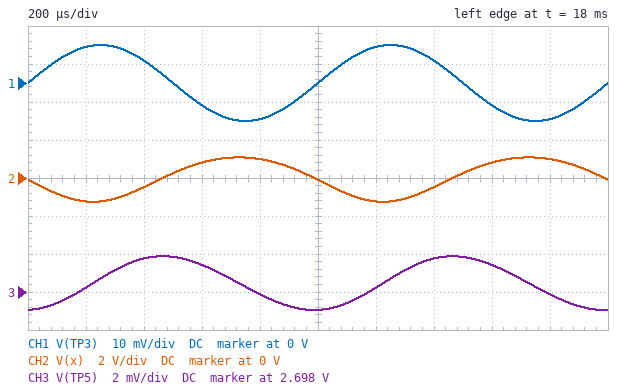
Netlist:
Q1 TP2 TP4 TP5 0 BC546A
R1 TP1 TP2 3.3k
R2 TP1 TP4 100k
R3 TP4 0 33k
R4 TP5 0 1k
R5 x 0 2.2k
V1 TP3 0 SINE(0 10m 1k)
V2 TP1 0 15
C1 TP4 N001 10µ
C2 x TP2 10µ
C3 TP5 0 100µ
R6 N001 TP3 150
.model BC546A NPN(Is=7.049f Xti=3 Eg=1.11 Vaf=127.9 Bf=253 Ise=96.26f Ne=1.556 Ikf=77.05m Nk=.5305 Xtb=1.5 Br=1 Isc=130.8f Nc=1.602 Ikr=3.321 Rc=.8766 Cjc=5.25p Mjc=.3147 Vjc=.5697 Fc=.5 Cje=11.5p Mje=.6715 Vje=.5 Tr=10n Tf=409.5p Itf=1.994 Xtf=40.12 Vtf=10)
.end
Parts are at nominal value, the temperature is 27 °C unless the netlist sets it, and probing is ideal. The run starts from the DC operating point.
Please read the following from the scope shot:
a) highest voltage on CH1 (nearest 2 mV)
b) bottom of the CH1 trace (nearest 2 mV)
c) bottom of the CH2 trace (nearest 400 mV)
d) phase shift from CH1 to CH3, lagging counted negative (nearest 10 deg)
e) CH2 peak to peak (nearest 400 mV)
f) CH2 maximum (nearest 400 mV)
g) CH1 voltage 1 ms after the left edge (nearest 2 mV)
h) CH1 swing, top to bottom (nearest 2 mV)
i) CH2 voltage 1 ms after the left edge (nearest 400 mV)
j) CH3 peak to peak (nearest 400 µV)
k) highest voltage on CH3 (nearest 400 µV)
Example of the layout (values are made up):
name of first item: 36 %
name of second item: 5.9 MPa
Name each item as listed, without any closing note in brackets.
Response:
highest voltage on CH1: 10 mV
bottom of the CH1 trace: -10 mV
bottom of the CH2 trace: -1.2 V
phase shift from CH1 to CH3, lagging counted negative: -80 deg
CH2 peak to peak: 2.4 V
CH2 maximum: 1.2 V
CH1 voltage 1 ms after the left edge: 0 V
CH1 swing, top to bottom: 20 mV
CH2 voltage 1 ms after the left edge: 0 V
CH3 peak to peak: 2.8 mV
highest voltage on CH3: 2.7000 V
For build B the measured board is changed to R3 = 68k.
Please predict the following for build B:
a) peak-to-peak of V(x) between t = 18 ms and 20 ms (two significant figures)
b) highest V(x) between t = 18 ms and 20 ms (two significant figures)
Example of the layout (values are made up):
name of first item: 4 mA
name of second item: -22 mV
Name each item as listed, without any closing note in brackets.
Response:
peak-to-peak of V(x) between t = 18 ms and 20 ms: 760 mV
highest V(x) between t = 18 ms and 20 ms: 640 mV
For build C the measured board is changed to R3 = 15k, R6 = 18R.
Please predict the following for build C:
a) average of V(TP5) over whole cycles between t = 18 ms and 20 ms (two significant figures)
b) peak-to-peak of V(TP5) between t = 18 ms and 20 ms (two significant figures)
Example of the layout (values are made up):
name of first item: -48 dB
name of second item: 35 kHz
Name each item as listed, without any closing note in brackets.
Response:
average of V(TP5) over whole cycles between t = 18 ms and 20 ms: 1.2 V
peak-to-peak of V(TP5) between t = 18 ms and 20 ms: 1.4 mV
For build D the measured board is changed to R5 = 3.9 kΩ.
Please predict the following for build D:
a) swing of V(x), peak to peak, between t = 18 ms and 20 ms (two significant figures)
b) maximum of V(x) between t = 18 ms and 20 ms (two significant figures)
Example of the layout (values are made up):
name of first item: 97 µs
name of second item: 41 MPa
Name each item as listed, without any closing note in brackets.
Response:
swing of V(x), peak to peak, between t = 18 ms and 20 ms: 3.1 V
maximum of V(x) between t = 18 ms and 20 ms: 1.5 V
